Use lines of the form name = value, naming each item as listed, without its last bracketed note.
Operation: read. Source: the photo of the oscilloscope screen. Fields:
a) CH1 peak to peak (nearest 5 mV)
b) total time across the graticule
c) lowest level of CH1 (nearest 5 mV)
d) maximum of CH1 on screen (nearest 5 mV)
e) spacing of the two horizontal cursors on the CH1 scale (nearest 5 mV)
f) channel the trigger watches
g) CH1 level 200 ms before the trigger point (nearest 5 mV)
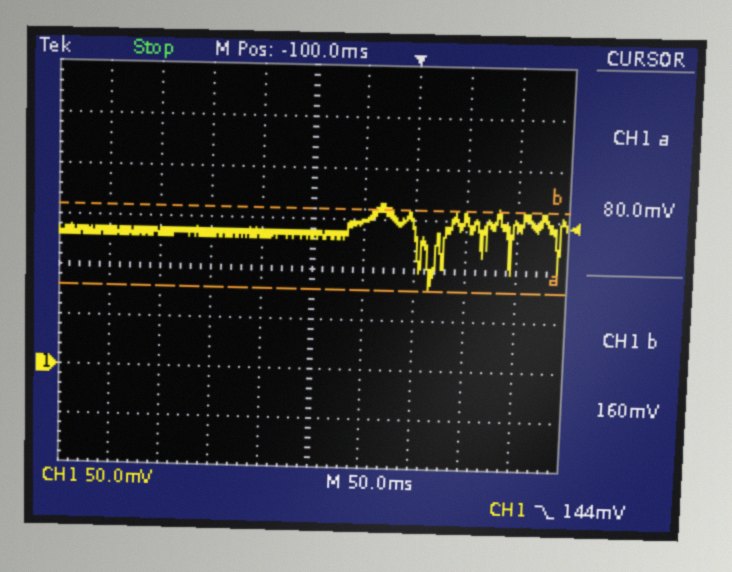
CH1 peak to peak = 80 mV
total time across the graticule = 500 ms
lowest level of CH1 = 85 mV
maximum of CH1 on screen = 165 mV
spacing of the two horizontal cursors on the CH1 scale = 80 mV
channel the trigger watches = CH1
CH1 level 200 ms before the trigger point = 135 mV
